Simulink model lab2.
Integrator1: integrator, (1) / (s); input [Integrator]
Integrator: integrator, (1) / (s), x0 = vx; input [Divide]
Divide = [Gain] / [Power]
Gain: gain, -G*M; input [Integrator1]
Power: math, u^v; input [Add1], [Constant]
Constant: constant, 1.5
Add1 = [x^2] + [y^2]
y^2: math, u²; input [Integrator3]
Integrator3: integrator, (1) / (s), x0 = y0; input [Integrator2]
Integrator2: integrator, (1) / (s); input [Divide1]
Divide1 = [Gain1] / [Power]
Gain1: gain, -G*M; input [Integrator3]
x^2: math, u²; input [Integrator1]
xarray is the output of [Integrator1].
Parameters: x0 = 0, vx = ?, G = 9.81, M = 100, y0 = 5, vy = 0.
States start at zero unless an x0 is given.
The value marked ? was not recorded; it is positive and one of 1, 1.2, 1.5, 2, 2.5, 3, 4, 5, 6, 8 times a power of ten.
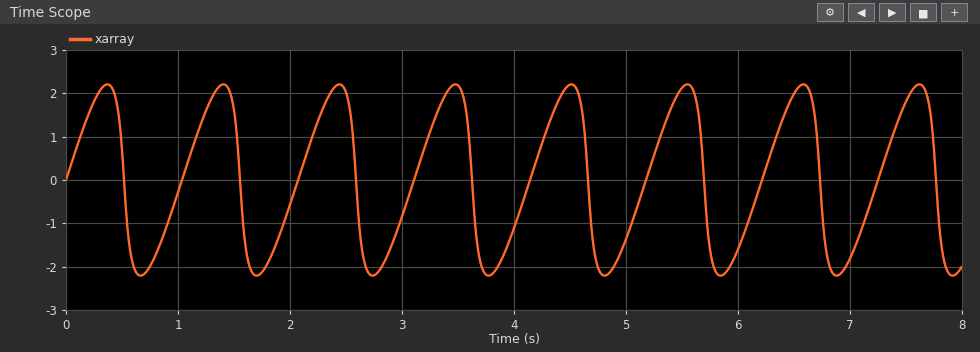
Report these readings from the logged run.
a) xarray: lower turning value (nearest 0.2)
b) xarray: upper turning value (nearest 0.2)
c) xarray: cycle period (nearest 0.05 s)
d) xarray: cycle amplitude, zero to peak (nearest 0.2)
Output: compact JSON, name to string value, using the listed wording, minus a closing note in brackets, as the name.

{"xarray: lower turning value": "-2.2", "xarray: upper turning value": "2.2", "xarray: cycle period": "1.05 s", "xarray: cycle amplitude, zero to peak": "2.2"}
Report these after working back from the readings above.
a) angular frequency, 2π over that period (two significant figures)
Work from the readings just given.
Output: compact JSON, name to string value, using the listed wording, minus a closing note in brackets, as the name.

{"angular frequency, 2π over that period": "6.0 rad/s"}
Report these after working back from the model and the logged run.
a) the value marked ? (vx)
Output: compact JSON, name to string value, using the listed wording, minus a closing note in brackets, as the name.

{"the value marked ?": "8"}
